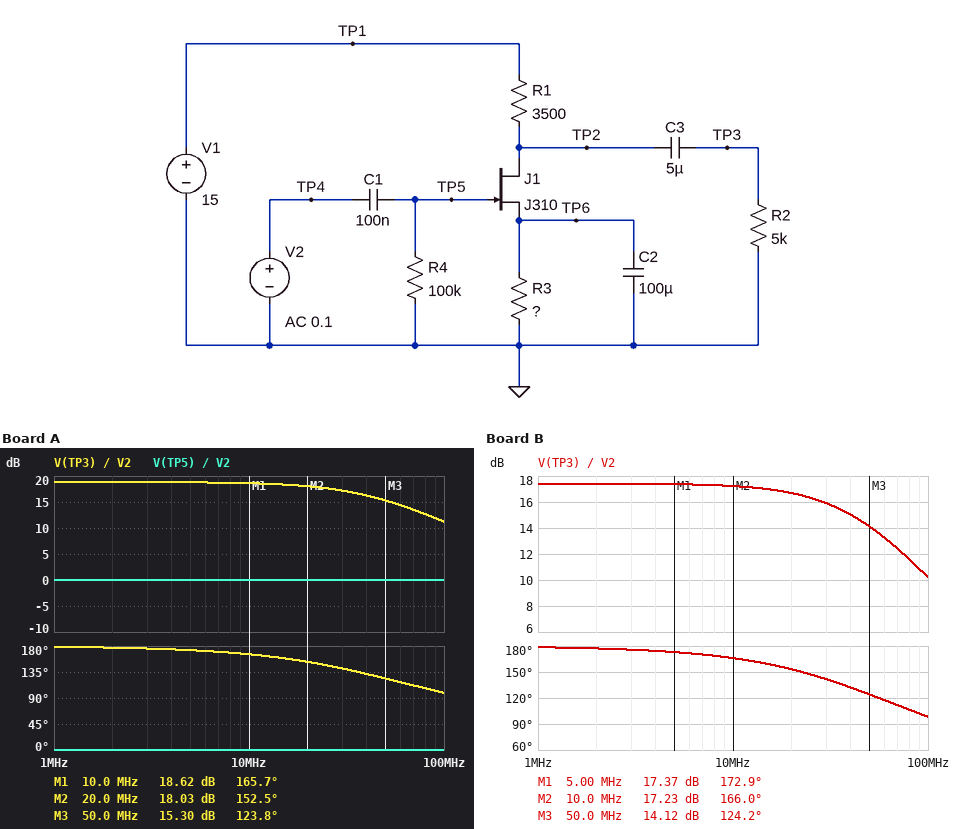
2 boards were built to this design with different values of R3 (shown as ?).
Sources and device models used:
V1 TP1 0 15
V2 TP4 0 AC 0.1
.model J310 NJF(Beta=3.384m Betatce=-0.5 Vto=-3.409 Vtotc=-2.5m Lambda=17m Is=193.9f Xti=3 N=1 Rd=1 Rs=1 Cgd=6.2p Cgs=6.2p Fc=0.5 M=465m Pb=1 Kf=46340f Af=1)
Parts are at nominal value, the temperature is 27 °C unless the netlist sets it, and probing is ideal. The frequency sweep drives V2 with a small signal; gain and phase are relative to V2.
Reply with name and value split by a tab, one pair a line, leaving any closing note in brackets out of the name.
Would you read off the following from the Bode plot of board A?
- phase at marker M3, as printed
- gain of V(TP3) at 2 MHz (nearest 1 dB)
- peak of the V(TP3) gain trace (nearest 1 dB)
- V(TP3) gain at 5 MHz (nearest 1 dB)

phase at marker M3, as printed	123.8 deg
gain of V(TP3) at 2 MHz	19 dB
peak of the V(TP3) gain trace	19 dB
V(TP3) gain at 5 MHz	19 dB
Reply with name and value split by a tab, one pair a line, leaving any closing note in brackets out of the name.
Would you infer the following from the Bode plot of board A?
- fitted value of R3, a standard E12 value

fitted value of R3, a standard E12 value	2.2 kΩ
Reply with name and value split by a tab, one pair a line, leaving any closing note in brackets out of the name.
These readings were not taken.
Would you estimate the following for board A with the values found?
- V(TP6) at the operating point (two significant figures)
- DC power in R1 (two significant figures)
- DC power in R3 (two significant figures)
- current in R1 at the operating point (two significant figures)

V(TP6) at the operating point	2.8 V
DC power in R1	5.8 mW
DC power in R3	3.6 mW
current in R1 at the operating point	1.3 mA
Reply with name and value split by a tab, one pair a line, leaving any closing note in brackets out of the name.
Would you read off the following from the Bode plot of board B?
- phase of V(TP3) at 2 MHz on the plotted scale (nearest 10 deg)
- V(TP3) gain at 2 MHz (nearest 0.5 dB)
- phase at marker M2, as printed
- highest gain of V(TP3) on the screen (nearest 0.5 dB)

phase of V(TP3) at 2 MHz on the plotted scale	180 deg
V(TP3) gain at 2 MHz	17.5 dB
phase at marker M2, as printed	166.0 deg
highest gain of V(TP3) on the screen	17.5 dB
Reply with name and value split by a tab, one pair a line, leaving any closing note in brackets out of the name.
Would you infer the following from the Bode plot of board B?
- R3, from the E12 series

R3, from the E12 series	3.3 kΩ
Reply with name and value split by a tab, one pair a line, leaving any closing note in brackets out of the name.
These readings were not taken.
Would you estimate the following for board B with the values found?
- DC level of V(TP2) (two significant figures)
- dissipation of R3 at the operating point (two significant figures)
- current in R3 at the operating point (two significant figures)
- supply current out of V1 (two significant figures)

DC level of V(TP2)	12 V
dissipation of R3 at the operating point	2.6 mW
current in R3 at the operating point	890 µA
supply current out of V1	890 µA
